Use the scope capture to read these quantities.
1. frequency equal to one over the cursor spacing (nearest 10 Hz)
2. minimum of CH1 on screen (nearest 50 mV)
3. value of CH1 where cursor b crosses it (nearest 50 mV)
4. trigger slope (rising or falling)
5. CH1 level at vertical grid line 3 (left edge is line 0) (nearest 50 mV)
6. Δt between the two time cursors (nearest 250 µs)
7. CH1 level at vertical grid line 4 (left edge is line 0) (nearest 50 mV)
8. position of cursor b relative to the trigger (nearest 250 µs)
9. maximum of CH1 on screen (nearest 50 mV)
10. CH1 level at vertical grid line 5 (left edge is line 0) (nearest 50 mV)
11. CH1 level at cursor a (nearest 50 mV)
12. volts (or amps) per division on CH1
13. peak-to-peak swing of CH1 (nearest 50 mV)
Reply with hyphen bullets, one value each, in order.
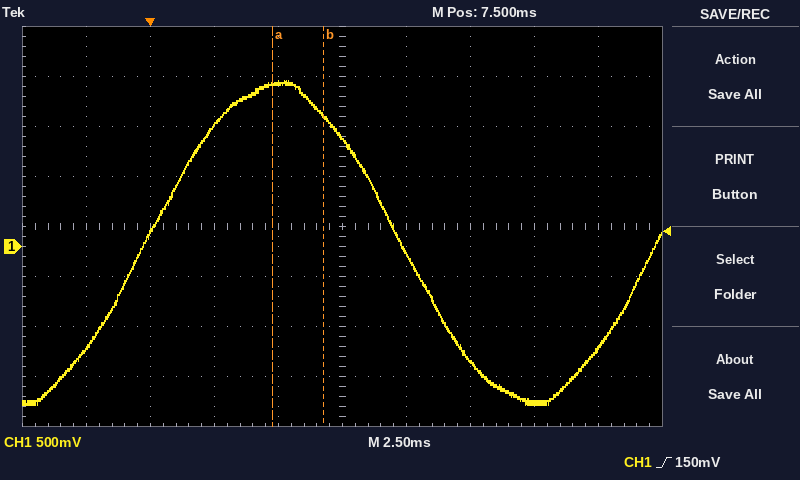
- 500 Hz
- -1.60 V
- 1.30 V
- rising
- 1.20 V
- 2.00 ms
- 1.65 V
- +6.75 ms
- 1.65 V
- 1.10 V
- 1.65 V
- 500 mV
- 3.25 V
